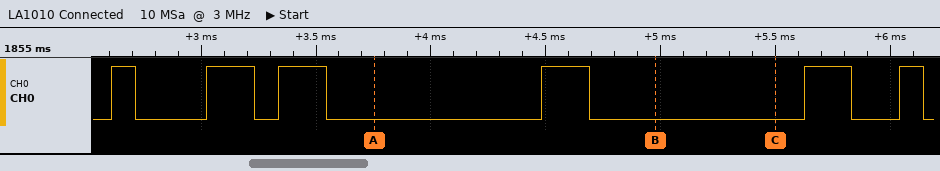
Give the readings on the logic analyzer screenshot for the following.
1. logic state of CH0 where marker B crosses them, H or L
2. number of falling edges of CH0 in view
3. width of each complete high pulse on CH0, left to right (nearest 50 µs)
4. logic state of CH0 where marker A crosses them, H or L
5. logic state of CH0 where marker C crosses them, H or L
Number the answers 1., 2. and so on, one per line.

1. CH0=L
2. 6
3. 100 µs, 200 µs, 200 µs, 200 µs, 200 µs, 100 µs
4. CH0=L
5. CH0=L
